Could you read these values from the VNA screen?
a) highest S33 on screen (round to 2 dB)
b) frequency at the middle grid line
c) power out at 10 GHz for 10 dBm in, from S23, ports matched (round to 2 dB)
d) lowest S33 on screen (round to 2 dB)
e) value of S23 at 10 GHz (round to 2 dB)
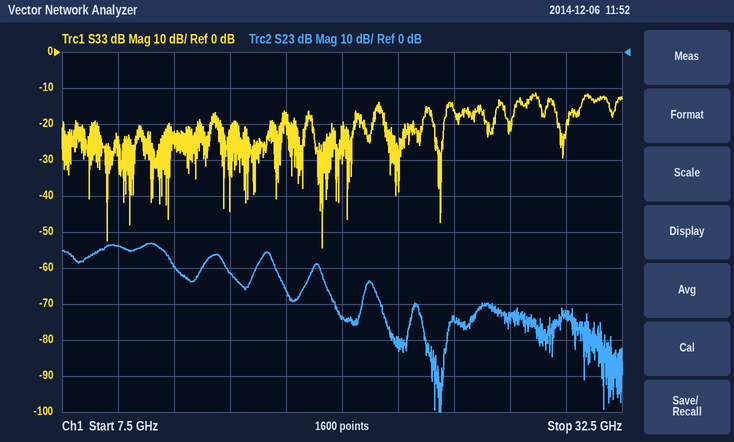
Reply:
-12 dB
20 GHz
-44 dBm
-54 dB
-54 dB
